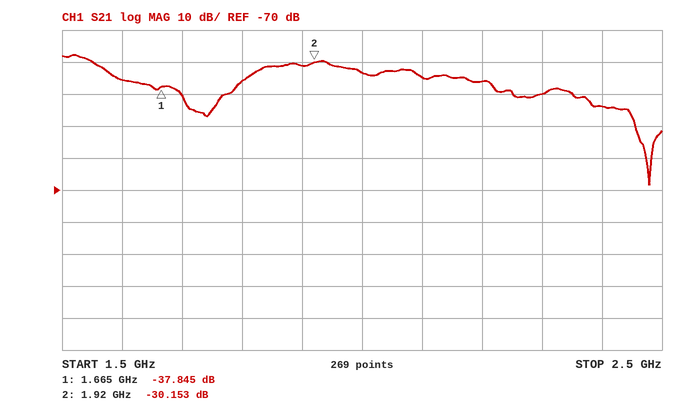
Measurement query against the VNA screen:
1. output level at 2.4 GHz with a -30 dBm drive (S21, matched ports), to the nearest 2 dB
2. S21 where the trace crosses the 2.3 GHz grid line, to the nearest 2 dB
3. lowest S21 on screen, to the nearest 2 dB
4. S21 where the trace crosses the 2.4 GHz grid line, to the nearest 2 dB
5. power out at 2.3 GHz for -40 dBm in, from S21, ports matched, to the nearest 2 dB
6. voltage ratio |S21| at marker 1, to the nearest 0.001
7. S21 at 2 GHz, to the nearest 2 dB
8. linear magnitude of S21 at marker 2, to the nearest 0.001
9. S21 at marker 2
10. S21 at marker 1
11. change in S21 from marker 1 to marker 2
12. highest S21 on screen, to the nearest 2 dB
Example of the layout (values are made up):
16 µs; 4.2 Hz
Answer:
-74 dBm; -40 dB; -68 dB; -44 dB; -80 dBm; 0.013; -34 dB; 0.031; -30.153 dB; -37.845 dB; 7.692 dB; -28 dB
